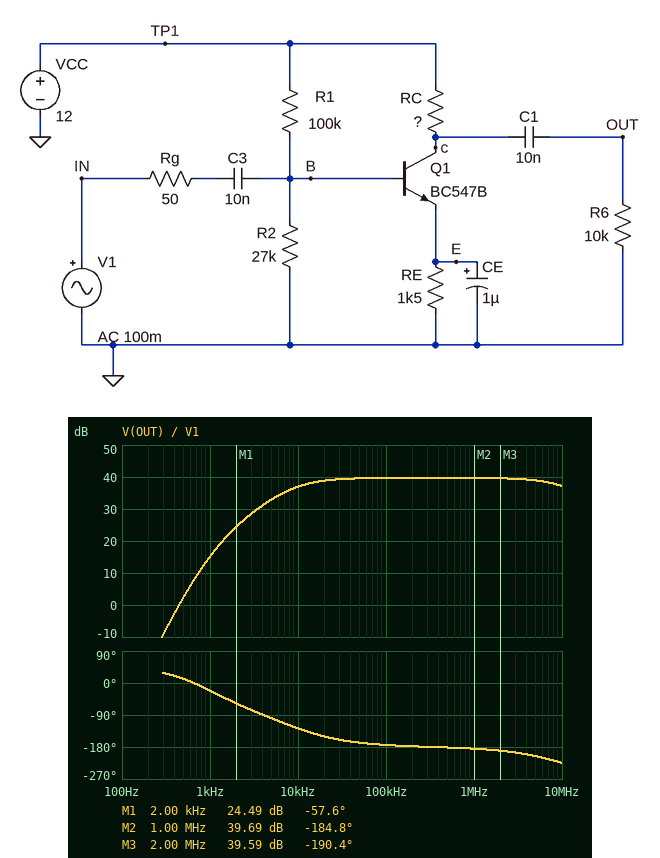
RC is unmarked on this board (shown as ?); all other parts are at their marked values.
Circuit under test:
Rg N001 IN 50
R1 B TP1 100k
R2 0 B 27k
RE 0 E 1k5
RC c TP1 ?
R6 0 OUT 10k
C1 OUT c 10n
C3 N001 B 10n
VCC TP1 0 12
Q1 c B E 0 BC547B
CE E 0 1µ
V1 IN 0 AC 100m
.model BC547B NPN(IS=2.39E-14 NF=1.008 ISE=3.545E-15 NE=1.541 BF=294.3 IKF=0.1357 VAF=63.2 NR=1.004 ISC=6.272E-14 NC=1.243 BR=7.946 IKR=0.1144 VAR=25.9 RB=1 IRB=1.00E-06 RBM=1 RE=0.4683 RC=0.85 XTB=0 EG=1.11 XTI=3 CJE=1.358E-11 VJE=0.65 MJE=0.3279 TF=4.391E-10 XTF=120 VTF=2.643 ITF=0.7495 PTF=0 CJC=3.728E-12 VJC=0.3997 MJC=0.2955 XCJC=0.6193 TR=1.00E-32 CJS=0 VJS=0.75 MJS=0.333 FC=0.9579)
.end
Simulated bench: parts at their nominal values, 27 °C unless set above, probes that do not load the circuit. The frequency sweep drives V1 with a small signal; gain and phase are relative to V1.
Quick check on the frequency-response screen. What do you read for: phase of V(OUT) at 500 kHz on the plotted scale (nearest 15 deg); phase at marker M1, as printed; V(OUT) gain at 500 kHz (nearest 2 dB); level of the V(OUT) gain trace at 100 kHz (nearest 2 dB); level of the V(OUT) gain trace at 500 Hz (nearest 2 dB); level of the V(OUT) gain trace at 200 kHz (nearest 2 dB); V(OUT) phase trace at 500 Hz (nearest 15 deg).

-180 deg
-57.6 deg
40 dB
40 dB
2 dB
40 dB
15 deg
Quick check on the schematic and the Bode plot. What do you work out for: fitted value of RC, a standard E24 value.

3 kΩ
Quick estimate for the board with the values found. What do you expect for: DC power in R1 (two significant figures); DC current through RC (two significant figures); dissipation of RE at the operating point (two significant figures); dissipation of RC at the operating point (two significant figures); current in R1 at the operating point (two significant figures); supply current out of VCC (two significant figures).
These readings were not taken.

910 µW
1.2 mA
2.2 mW
4.4 mW
95 µA
1.3 mA
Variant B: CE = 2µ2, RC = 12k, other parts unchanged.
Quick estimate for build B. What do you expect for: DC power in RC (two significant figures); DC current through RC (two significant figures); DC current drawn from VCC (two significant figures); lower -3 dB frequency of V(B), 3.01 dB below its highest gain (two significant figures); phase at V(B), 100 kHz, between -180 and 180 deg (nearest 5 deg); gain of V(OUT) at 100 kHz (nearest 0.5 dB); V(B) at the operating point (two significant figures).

9.3 mW
880 µA
980 µA
66 kHz
35 deg
11.0 dB
2.0 V
